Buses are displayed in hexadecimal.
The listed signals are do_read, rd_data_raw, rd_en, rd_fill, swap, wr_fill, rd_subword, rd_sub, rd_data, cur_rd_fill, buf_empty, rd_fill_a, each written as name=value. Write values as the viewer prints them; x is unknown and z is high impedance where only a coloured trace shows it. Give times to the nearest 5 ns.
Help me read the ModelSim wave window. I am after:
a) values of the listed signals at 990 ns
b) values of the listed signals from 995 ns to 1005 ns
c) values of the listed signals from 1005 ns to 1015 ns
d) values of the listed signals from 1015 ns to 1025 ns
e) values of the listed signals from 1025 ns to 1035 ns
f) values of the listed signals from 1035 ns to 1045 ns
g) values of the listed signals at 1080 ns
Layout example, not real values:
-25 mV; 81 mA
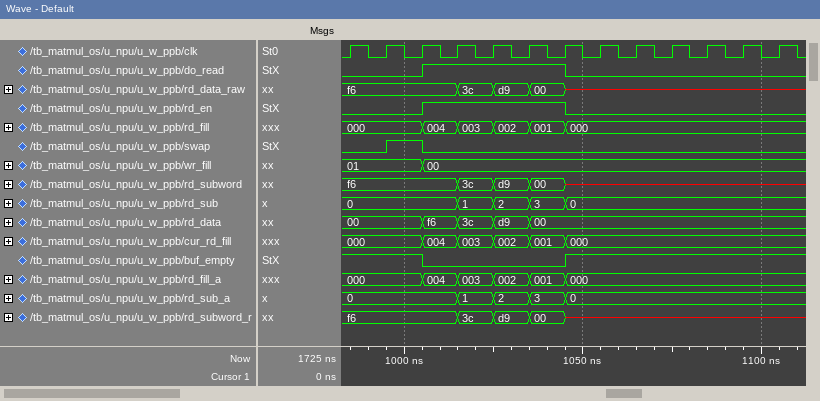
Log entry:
do_read=0, rd_data_raw=f6, rd_en=0, rd_fill=000, swap=0, wr_fill=01, rd_subword=f6, rd_sub=0, rd_data=00, cur_rd_fill=000, buf_empty=1, rd_fill_a=000; do_read=0, rd_data_raw=f6, rd_en=0, rd_fill=000, swap=1, wr_fill=01, rd_subword=f6, rd_sub=0, rd_data=00, cur_rd_fill=000, buf_empty=1, rd_fill_a=000; do_read=1, rd_data_raw=f6, rd_en=1, rd_fill=004, swap=0, wr_fill=00, rd_subword=f6, rd_sub=0, rd_data=f6, cur_rd_fill=004, buf_empty=0, rd_fill_a=004; do_read=1, rd_data_raw=3c, rd_en=1, rd_fill=003, swap=0, wr_fill=00, rd_subword=3c, rd_sub=1, rd_data=3c, cur_rd_fill=003, buf_empty=0, rd_fill_a=003; do_read=1, rd_data_raw=d9, rd_en=1, rd_fill=002, swap=0, wr_fill=00, rd_subword=d9, rd_sub=2, rd_data=d9, cur_rd_fill=002, buf_empty=0, rd_fill_a=002; do_read=1, rd_data_raw=00, rd_en=1, rd_fill=001, swap=0, wr_fill=00, rd_subword=00, rd_sub=3, rd_data=00, cur_rd_fill=001, buf_empty=0, rd_fill_a=001; do_read=0, rd_data_raw=x, rd_en=0, rd_fill=000, swap=0, wr_fill=00, rd_subword=x, rd_sub=0, rd_data=00, cur_rd_fill=000, buf_empty=1, rd_fill_a=000
